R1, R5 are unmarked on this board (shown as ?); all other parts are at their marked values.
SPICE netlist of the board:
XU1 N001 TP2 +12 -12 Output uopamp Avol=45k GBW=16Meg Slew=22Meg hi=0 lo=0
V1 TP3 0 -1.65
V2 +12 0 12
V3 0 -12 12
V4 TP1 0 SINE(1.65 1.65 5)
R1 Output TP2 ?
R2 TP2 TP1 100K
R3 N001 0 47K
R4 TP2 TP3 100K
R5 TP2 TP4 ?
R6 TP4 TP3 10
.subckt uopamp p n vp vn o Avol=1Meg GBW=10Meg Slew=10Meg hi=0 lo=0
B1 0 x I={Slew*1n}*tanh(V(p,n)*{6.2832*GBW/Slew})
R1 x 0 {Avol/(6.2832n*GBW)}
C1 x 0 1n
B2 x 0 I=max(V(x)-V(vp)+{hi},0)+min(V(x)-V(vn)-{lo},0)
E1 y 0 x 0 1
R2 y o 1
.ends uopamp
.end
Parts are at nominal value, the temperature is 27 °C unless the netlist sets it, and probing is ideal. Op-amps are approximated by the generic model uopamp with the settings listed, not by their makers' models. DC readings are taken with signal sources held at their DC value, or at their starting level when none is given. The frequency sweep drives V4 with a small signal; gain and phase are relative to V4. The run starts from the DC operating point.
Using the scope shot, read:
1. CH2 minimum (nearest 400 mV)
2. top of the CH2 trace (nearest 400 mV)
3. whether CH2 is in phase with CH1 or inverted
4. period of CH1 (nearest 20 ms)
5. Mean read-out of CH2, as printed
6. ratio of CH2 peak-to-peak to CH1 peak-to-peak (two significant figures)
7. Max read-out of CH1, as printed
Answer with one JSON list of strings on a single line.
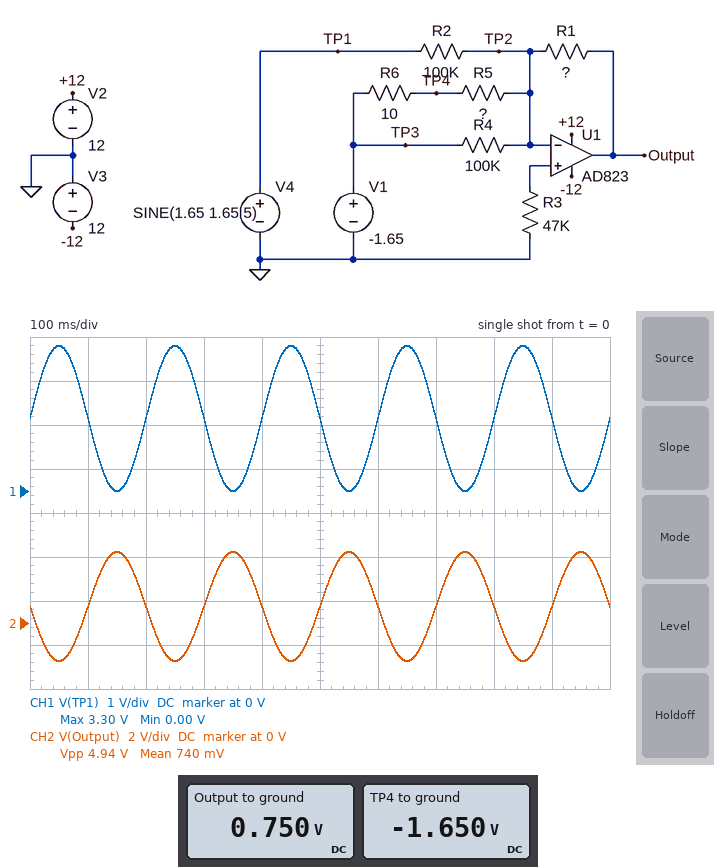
["-1.6 V", "3.2 V", "inverted", "200 ms", "740 mV", "1.5", "3.30 V"]
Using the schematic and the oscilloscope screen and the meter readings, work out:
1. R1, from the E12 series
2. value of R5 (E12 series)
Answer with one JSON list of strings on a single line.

["150 kΩ", "330 kΩ"]
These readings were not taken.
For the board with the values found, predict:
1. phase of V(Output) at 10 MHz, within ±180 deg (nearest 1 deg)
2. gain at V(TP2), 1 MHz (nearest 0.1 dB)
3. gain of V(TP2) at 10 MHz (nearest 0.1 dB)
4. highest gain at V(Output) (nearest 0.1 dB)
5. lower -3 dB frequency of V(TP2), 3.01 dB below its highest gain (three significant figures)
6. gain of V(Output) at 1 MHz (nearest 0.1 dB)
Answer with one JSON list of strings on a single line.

["110 deg", "-20.9 dB", "-10.0 dB", "3.5 dB", "3.59 MHz", "3.2 dB"]
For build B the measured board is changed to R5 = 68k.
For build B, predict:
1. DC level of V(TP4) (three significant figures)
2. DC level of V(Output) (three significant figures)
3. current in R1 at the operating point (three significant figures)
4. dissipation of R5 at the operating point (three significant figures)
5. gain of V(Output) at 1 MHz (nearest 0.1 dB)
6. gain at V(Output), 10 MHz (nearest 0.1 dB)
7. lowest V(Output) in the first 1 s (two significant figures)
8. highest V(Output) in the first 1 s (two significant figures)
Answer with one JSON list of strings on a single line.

["-1.65 V", "3.64 V", "24.3 µA", "40.0 µW", "2.9 dB", "-8.5 dB", "1.2 V", "6.1 V"]
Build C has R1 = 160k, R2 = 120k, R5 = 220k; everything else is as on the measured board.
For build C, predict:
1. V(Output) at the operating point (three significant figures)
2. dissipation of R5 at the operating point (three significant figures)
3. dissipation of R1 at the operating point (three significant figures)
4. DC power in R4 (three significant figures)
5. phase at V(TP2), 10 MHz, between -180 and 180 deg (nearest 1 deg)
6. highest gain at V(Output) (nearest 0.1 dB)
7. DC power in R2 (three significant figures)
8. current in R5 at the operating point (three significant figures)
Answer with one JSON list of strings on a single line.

["1.64 V", "12.4 µW", "16.8 µW", "27.2 µW", "19 deg", "2.5 dB", "22.7 µW", "7.50 µA"]
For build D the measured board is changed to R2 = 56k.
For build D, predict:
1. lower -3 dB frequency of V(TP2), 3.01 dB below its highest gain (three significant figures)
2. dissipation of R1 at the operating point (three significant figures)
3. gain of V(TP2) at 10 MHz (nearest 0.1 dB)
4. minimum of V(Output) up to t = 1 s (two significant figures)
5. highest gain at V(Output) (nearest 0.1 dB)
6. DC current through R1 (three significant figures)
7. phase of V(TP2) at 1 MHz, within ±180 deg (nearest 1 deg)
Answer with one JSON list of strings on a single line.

["2.84 MHz", "9.51 µW", "-6.8 dB", "-5.6 V", "8.6 dB", "7.96 µA", "71 deg"]
